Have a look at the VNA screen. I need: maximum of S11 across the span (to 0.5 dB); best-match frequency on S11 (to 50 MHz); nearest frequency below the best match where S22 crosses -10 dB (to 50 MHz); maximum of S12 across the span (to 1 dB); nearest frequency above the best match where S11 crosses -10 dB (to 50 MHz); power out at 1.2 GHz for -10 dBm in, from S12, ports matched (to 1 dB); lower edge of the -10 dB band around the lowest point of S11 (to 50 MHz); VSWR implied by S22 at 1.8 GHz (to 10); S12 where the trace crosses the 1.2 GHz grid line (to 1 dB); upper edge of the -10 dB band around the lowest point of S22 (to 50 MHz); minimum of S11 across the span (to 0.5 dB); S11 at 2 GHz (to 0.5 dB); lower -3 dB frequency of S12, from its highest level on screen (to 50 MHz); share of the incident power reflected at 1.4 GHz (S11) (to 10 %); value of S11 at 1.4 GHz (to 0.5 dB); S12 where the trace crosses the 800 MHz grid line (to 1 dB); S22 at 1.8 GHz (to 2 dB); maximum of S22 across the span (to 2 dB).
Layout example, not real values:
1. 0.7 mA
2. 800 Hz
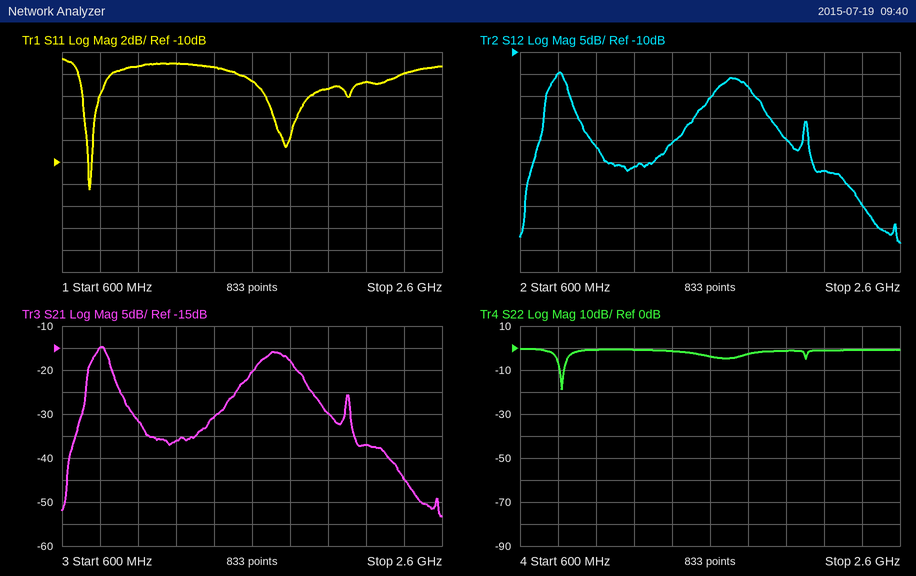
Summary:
1. -0.5 dB
2. 750 MHz
3. 800 MHz
4. -15 dB
5. 750 MHz
6. -46 dBm
7. 750 MHz
8. 10
9. -36 dB
10. 850 MHz
11. -12.5 dB
12. -3.5 dB
13. 750 MHz
14. 70 %
15. -1.5 dB
16. -15 dB
17. -2 dB
18. 0 dB
